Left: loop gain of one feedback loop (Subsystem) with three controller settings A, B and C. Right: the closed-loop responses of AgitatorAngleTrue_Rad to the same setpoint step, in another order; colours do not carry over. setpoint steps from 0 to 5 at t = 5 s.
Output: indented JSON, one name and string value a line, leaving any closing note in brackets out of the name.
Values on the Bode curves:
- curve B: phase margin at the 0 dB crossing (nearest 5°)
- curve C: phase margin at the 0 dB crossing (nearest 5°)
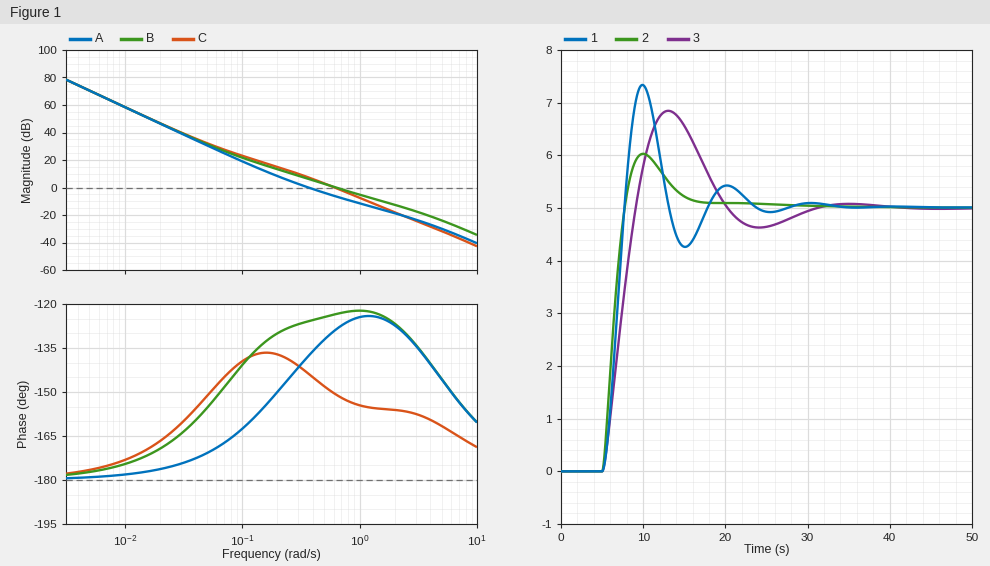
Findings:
{
  "curve B: phase margin at the 0 dB crossing": "55°",
  "curve C: phase margin at the 0 dB crossing": "30°"
}
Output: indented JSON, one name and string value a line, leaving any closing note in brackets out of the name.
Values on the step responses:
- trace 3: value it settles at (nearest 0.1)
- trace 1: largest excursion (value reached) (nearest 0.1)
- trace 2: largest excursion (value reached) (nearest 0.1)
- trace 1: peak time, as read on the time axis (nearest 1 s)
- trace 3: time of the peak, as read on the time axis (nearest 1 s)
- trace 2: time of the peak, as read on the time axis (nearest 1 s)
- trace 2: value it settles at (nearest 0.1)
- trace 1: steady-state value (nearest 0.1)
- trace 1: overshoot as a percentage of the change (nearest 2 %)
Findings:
{
  "trace 3: value it settles at": "5.0",
  "trace 1: largest excursion (value reached)": "7.3",
  "trace 2: largest excursion (value reached)": "6.0",
  "trace 1: peak time, as read on the time axis": "10 s",
  "trace 3: time of the peak, as read on the time axis": "13 s",
  "trace 2: time of the peak, as read on the time axis": "10 s",
  "trace 2: value it settles at": "5.0",
  "trace 1: steady-state value": "5.0",
  "trace 1: overshoot as a percentage of the change": "46 %"
}
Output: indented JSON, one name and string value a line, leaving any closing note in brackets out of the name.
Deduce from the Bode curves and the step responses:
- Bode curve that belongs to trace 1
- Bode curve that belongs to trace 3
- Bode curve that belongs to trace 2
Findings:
{
  "Bode curve that belongs to trace 1": "C",
  "Bode curve that belongs to trace 3": "A",
  "Bode curve that belongs to trace 2": "B"
}
